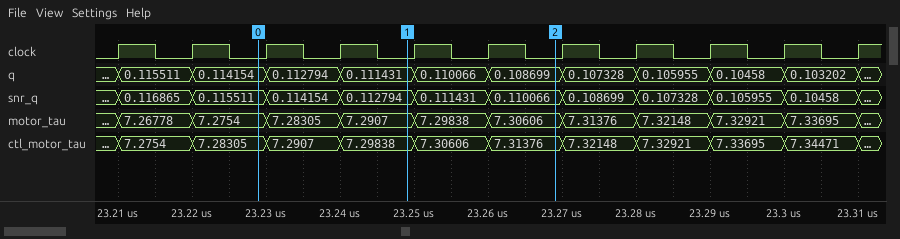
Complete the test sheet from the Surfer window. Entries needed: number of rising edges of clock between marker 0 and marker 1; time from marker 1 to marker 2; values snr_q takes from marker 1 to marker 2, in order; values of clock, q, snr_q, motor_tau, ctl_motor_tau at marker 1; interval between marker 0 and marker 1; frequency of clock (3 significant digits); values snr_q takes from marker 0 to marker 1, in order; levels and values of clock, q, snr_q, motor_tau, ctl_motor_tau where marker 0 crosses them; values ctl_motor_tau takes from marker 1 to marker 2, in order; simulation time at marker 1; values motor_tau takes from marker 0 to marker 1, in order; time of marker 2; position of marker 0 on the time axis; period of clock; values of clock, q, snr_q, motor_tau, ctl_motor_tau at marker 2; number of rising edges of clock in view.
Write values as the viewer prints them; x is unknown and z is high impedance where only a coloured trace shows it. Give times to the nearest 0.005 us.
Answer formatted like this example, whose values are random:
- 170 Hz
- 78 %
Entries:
- 2
- 0.02 us
- 0.112794, 0.111431, 0.110066
- clock=0, q=0.111431, snr_q=0.112794, motor_tau=7.2907, ctl_motor_tau=7.29838
- 0.02 us
- 100 MHz
- 0.115511, 0.114154, 0.112794
- clock=0, q=0.114154, snr_q=0.115511, motor_tau=7.2754, ctl_motor_tau=7.28305
- 7.29838, 7.30606, 7.31376
- 23.25 us
- 7.2754, 7.28305, 7.2907
- 23.27 us
- 23.23 us
- 0.01 us
- clock=0, q=0.108699, snr_q=0.110066, motor_tau=7.30606, ctl_motor_tau=7.31376
- 11
